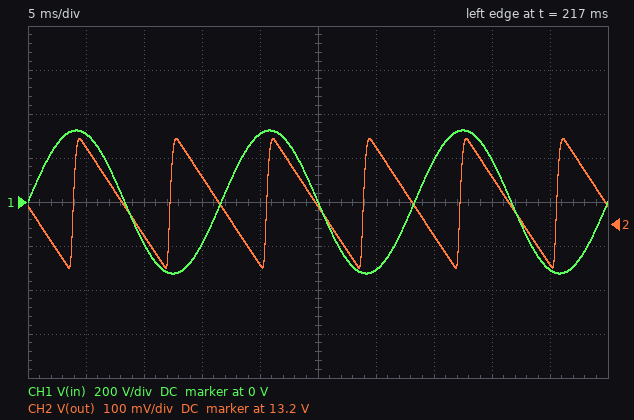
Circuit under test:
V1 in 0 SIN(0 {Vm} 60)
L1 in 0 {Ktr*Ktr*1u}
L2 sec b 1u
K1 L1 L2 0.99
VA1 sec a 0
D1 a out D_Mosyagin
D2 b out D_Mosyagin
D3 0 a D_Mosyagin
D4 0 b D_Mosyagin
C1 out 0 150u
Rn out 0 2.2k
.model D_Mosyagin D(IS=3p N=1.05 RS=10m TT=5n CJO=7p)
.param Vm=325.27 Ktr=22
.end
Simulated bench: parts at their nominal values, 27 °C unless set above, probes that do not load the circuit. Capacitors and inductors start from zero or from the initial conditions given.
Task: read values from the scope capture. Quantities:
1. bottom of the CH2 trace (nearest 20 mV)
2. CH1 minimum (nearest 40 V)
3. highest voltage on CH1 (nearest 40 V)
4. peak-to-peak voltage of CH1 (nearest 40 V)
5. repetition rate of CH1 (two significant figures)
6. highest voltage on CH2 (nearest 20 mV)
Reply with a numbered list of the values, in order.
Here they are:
1. 13.10 V
2. -320 V
3. 320 V
4. 640 V
5. 60 Hz
6. 13.40 V
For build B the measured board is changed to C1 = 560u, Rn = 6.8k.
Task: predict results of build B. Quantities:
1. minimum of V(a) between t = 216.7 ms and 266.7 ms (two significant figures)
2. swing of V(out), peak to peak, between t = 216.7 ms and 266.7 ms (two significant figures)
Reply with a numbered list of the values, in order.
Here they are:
1. -630 mV
2. 26 mV
